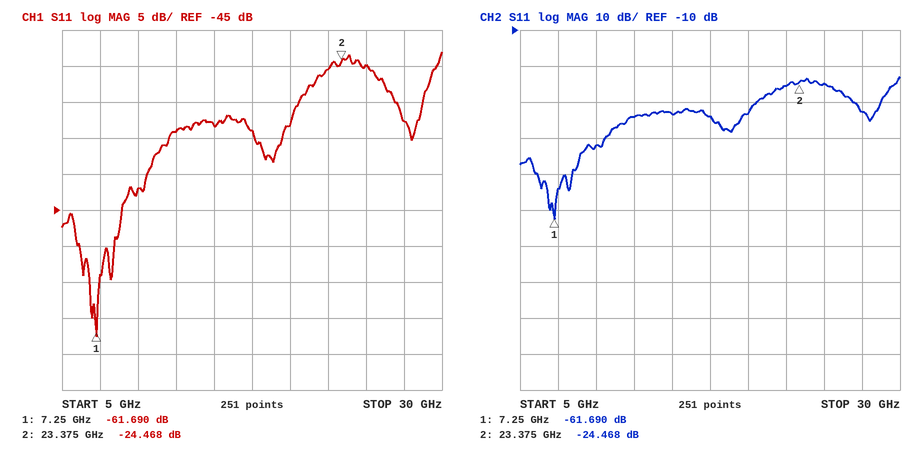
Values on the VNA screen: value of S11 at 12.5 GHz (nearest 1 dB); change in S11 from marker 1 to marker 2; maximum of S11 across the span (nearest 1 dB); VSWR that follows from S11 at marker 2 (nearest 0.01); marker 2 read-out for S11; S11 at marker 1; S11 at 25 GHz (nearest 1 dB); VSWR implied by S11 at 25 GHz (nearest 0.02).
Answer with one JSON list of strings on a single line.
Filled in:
["-34 dB", "37.222 dB", "-23 dB", "1.13", "-24.468 dB", "-61.690 dB", "-25 dB", "1.12"]
